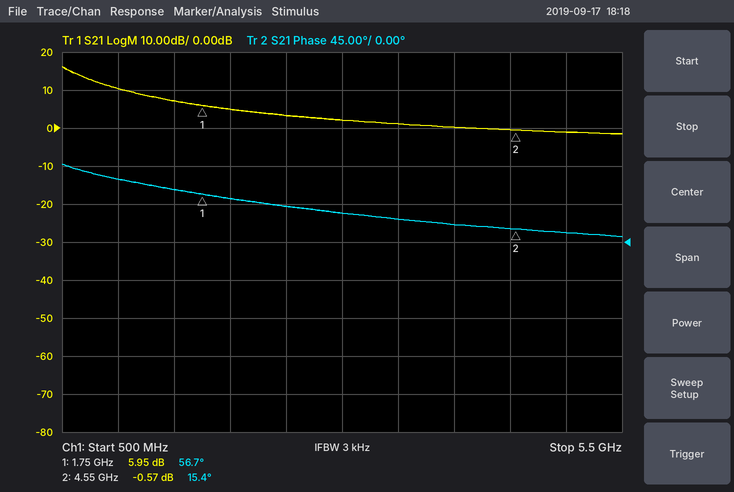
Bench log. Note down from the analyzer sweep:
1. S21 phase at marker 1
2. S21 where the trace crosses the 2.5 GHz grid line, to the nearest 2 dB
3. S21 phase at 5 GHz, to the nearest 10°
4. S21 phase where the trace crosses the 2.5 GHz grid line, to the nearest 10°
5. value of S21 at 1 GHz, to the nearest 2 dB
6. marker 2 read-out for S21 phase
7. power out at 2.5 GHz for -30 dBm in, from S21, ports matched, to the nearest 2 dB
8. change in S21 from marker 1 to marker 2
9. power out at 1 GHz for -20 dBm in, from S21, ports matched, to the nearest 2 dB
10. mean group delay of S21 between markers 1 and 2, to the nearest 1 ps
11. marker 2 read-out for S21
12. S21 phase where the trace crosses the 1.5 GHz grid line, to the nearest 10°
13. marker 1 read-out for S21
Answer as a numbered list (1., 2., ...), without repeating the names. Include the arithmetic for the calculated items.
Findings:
1. 56.7°
2. 4 dB
3. 10°
4. 40°
5. 10 dB
6. 15.4°
7. -30 dBm + (4 dB) = -26 dBm
8. -0.57 − (5.95) = -6.52 dB
9. -20 dBm + (10 dB) = -10 dBm
10. −(15.4° − (56.7°))/(360° × 2.8 GHz) ≈ 41 ps
11. -0.57 dB
12. 60°
13. 5.95 dB
